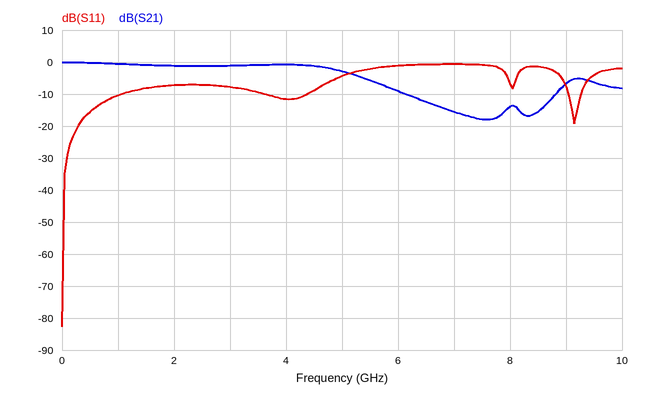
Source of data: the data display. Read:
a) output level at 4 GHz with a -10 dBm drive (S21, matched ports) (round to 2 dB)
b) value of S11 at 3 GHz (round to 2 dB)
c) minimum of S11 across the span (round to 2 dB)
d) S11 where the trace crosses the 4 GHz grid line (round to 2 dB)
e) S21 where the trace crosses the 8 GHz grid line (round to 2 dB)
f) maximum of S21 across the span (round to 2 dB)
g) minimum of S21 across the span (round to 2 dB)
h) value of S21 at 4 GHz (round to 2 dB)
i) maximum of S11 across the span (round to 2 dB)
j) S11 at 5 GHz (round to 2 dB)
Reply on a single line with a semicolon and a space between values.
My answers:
-10 dBm; -8 dB; -82 dB; -12 dB; -14 dB; 0 dB; -18 dB; 0 dB; 0 dB; -4 dB
